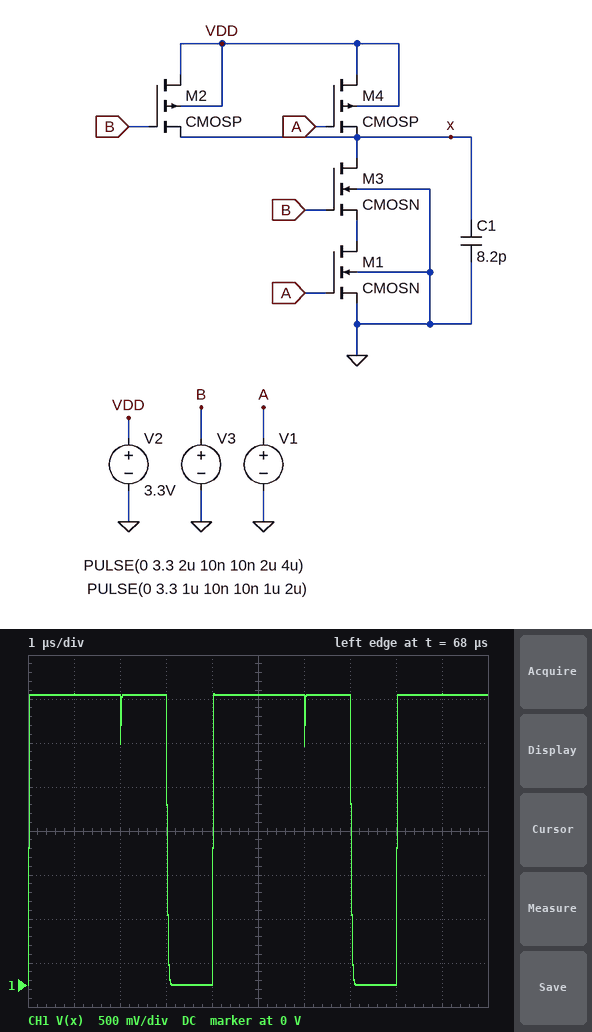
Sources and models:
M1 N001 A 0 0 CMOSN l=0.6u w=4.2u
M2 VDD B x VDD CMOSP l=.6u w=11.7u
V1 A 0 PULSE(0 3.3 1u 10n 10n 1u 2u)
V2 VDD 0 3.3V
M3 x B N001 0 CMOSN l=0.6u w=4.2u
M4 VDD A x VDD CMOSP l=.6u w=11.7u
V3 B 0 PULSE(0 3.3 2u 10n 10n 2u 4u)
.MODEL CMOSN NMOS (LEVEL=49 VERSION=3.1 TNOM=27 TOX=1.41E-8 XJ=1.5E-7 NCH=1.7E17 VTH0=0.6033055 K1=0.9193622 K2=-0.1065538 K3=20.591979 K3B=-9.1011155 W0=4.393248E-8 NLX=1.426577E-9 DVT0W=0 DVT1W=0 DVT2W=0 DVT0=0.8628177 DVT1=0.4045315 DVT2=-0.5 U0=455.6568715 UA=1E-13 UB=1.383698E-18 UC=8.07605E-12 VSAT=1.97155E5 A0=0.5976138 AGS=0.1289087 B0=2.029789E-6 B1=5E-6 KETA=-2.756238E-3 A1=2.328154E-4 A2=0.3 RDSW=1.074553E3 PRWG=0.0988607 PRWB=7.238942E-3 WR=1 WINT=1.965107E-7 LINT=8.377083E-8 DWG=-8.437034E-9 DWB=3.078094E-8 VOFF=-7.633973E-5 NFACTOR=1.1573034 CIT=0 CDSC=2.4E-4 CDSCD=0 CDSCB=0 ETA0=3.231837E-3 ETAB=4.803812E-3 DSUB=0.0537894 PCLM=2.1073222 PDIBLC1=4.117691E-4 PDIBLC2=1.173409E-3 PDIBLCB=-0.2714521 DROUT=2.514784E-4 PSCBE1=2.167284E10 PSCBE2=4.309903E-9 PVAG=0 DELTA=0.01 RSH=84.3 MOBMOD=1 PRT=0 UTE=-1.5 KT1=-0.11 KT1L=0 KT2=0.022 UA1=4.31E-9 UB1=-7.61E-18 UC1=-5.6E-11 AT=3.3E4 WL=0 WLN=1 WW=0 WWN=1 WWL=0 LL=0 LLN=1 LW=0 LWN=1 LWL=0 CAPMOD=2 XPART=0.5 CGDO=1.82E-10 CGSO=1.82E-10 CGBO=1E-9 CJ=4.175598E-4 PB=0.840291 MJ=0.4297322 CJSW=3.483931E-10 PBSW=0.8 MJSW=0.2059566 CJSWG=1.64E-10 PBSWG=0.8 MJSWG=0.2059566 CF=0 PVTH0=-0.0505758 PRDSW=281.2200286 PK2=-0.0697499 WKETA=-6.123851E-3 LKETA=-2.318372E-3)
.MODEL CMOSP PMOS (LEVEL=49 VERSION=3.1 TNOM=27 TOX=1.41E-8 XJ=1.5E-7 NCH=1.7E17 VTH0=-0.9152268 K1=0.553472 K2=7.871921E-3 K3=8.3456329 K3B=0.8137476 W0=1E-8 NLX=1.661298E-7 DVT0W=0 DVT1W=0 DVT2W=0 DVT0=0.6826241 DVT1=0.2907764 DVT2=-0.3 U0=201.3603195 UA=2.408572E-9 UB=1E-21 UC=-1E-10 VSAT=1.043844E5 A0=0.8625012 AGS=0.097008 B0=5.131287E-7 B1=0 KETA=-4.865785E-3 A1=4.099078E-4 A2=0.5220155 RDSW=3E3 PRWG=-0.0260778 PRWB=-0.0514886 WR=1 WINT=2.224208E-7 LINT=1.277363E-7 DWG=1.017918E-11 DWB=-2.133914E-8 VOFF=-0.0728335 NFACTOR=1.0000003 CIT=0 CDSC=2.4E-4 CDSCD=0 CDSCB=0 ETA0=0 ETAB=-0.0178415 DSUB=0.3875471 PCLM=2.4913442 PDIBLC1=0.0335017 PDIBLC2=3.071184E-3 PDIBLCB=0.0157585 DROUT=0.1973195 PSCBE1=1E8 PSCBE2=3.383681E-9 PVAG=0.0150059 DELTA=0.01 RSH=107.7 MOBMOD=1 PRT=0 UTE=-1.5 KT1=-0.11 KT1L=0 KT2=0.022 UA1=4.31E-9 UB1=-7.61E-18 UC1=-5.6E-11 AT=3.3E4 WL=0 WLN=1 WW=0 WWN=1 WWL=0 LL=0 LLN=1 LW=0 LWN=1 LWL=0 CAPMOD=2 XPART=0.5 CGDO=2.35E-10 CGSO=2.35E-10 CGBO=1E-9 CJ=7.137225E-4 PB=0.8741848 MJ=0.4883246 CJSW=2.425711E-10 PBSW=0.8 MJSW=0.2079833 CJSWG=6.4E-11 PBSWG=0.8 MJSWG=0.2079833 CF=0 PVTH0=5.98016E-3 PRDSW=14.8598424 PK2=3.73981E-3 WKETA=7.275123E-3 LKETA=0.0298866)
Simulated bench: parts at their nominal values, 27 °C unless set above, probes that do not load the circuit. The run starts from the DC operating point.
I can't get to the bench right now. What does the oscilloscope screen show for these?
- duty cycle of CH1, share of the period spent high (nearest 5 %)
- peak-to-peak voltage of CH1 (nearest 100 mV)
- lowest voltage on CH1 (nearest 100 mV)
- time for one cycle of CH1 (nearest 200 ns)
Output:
75 %
3.3 V
0 V
4.0 µs
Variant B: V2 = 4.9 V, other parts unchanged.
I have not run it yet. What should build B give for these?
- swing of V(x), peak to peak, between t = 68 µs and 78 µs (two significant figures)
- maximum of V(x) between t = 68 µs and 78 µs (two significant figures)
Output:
3.6 V
4.9 V
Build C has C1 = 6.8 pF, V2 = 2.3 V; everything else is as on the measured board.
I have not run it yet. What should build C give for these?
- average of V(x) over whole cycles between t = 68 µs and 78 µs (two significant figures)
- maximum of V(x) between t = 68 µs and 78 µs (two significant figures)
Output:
1.7 V
2.3 V
